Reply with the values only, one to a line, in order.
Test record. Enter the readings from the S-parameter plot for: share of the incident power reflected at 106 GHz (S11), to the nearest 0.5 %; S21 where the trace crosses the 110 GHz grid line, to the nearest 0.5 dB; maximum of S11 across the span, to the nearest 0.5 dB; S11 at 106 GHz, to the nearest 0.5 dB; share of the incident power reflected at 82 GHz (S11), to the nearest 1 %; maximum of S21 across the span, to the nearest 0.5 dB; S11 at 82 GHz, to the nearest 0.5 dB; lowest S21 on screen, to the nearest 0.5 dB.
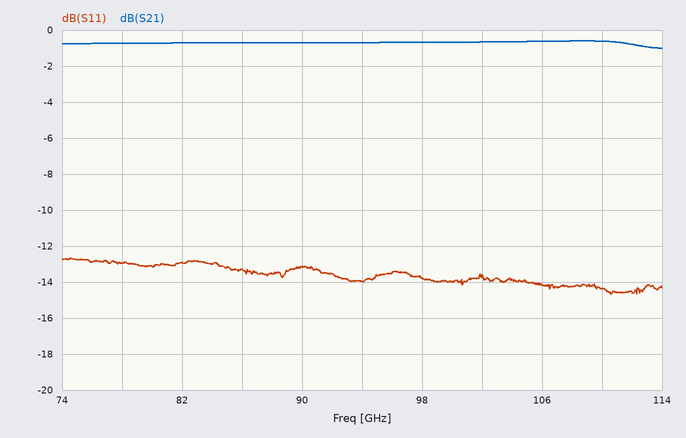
4.0 %
-0.5 dB
-12.5 dB
-14.0 dB
5 %
-0.5 dB
-13.0 dB
-1.0 dB
